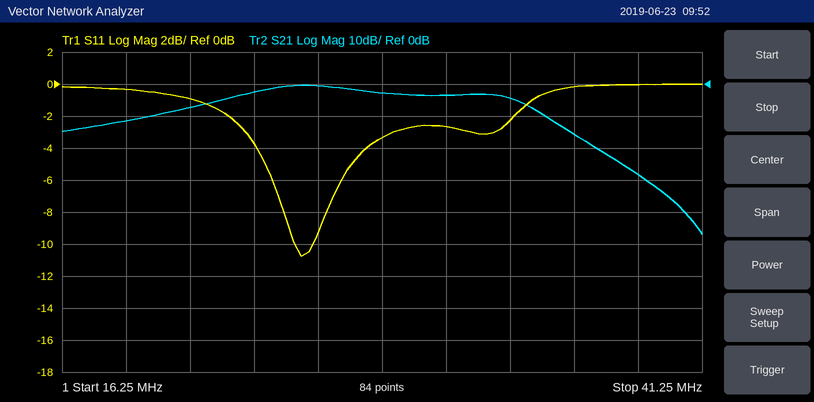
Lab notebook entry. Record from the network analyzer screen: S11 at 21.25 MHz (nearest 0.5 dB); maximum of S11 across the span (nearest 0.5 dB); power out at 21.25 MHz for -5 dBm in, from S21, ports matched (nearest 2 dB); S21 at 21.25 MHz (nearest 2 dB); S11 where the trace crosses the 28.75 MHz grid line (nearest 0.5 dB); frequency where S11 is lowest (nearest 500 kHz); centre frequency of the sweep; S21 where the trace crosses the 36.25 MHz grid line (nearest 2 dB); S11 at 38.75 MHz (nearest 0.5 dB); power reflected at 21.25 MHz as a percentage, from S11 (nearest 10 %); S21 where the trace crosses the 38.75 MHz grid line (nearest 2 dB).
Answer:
-1.0 dB
0.0 dB
-12 dBm
-8 dB
-3.5 dB
25.5 MHz
28.75 MHz
-16 dB
0.0 dB
80 %
-28 dB
